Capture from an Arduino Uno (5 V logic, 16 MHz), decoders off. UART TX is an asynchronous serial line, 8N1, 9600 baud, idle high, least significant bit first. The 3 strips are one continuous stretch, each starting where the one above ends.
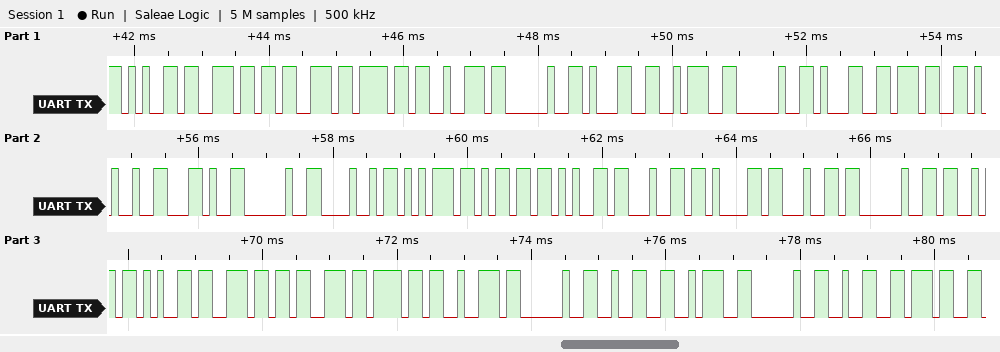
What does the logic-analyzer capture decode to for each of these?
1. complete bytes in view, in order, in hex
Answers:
65 6E 73 6F 72 20 31 3A 20 31 37 25 2C 20 48 75 6D 65 64 61 64 20 53 65 6E 73 6F 72 20 32 3A 20 32 37
